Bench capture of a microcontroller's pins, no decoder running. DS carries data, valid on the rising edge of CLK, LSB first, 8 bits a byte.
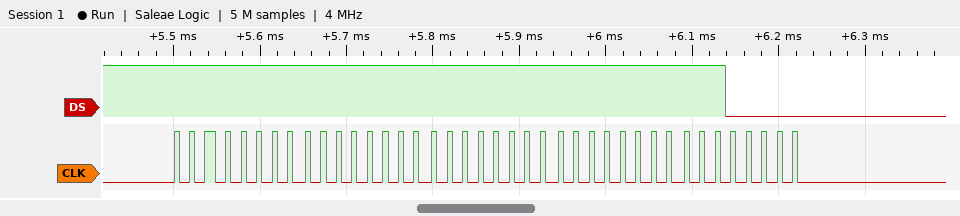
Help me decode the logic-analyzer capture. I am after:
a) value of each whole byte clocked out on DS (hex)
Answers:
FF FF FF FF 07
